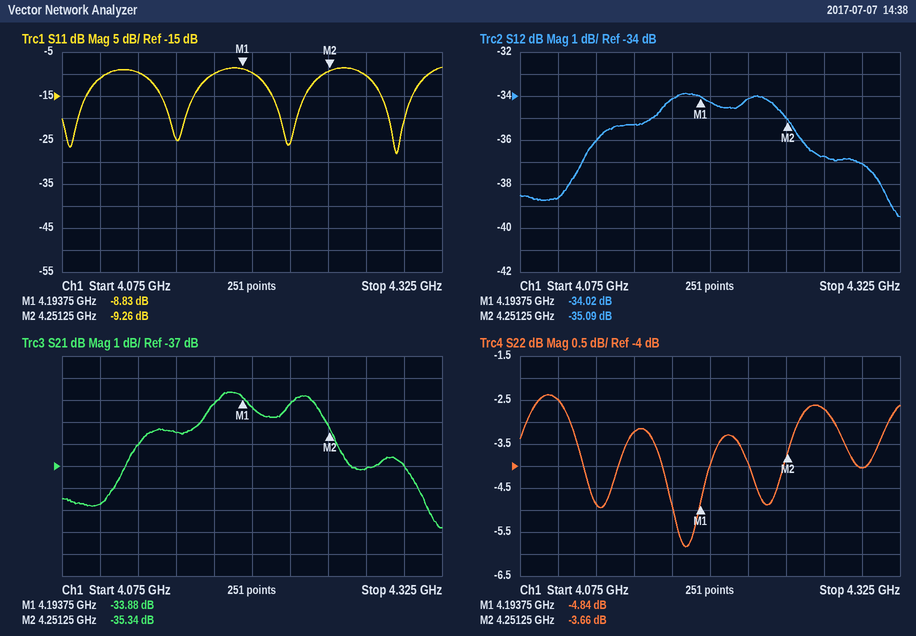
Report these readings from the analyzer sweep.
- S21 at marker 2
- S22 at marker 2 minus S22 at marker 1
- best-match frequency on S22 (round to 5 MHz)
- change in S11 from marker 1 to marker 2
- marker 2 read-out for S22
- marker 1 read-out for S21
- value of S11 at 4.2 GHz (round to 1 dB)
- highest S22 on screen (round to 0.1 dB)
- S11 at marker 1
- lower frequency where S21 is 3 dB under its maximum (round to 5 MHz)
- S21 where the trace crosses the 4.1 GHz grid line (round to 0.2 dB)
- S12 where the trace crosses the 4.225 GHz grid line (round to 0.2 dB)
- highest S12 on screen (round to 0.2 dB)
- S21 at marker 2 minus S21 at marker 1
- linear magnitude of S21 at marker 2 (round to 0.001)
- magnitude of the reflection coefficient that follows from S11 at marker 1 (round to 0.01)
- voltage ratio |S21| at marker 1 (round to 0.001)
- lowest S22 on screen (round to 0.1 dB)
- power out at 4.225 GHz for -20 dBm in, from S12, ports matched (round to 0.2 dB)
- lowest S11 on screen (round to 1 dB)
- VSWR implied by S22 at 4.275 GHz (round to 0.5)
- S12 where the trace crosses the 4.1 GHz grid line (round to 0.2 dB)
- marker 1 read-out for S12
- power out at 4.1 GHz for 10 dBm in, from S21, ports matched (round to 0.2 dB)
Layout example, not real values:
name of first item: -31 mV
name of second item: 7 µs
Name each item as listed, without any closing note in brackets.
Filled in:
S21 at marker 2: -35.34 dB
S22 at marker 2 minus S22 at marker 1: 1.18 dB
best-match frequency on S22: 4.185 GHz
change in S11 from marker 1 to marker 2: -0.43 dB
marker 2 read-out for S22: -3.66 dB
marker 1 read-out for S21: -33.88 dB
value of S11 at 4.2 GHz: -10 dB
highest S22 on screen: -2.4 dB
S11 at marker 1: -8.83 dB
lower frequency where S21 is 3 dB under its maximum: 4.120 GHz
S21 where the trace crosses the 4.1 GHz grid line: -38.8 dB
S12 where the trace crosses the 4.225 GHz grid line: -34.2 dB
highest S12 on screen: -33.8 dB
S21 at marker 2 minus S21 at marker 1: -1.46 dB
linear magnitude of S21 at marker 2: 0.017
magnitude of the reflection coefficient that follows from S11 at marker 1: 0.36
voltage ratio |S21| at marker 1: 0.020
lowest S22 on screen: -5.8 dB
power out at 4.225 GHz for -20 dBm in, from S12, ports matched: -54.2 dBm
lowest S11 on screen: -28 dB
VSWR implied by S22 at 4.275 GHz: 6.5
S12 where the trace crosses the 4.1 GHz grid line: -38.6 dB
marker 1 read-out for S12: -34.02 dB
power out at 4.1 GHz for 10 dBm in, from S21, ports matched: -28.8 dBm
